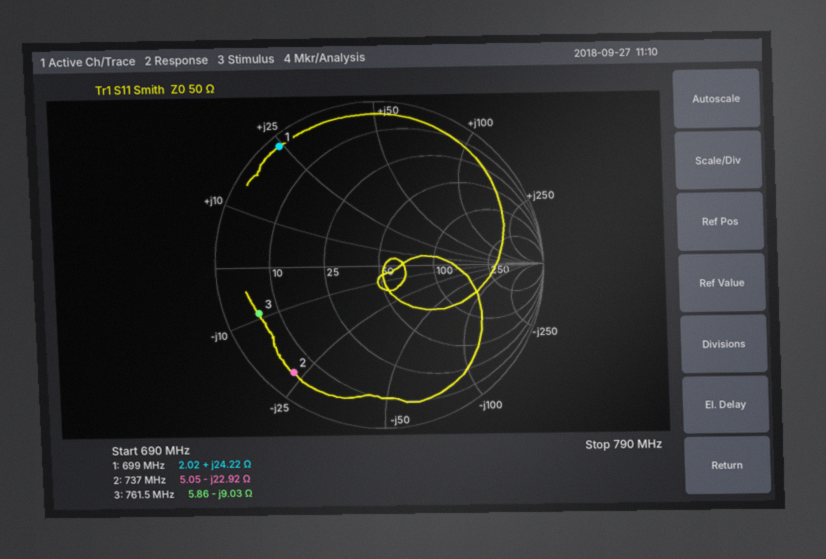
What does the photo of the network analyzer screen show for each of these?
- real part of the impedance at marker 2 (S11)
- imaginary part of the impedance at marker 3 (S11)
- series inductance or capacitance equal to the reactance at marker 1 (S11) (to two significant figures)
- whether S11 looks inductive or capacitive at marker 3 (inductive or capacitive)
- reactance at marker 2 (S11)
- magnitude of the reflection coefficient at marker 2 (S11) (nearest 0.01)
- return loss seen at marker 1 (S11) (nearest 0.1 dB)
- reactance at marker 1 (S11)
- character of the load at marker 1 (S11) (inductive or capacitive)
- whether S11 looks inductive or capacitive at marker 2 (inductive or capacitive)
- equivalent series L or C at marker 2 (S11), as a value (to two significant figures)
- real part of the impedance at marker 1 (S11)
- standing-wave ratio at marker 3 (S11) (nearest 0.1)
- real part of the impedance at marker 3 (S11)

5.05 Ω
-9.03 Ω
5.5 nH
capacitive
-22.92 Ω
0.85
0.6 dB
+24.22 Ω
inductive
capacitive
9.4 pF
2.02 Ω
8.8
5.86 Ω
